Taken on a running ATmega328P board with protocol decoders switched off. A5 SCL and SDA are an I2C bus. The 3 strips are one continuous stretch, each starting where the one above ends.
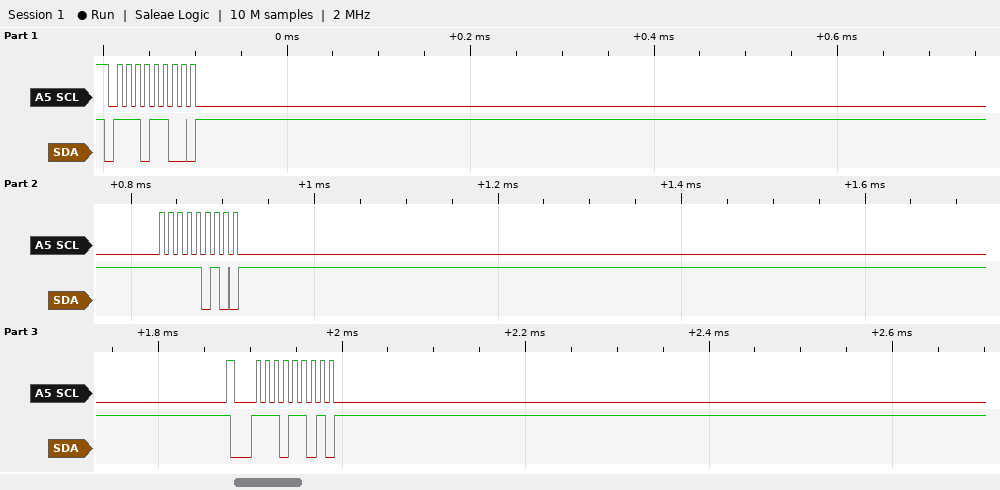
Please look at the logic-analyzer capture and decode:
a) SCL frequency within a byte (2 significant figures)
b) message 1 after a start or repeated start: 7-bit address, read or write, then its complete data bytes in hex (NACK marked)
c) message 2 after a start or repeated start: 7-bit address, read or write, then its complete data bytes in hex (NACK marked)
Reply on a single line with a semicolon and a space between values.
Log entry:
100 kHz; 0x76 write: FA; 0x76 read
